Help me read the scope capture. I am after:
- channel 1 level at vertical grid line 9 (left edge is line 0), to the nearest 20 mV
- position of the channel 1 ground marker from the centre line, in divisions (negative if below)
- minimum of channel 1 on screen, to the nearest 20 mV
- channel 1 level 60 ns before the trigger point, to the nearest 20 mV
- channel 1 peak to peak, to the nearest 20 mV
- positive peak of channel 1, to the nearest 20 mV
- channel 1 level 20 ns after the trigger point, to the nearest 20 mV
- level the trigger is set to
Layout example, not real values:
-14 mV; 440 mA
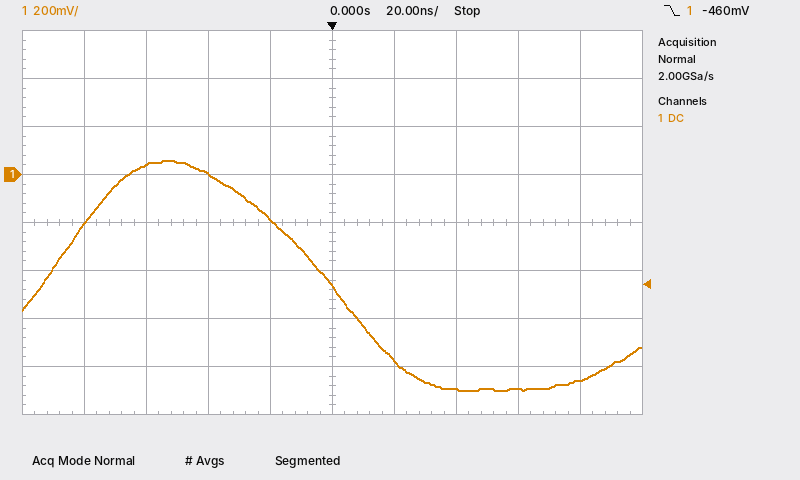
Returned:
-860 mV; +1.0 div; -900 mV; 40 mV; 960 mV; 60 mV; -780 mV; -460 mV
